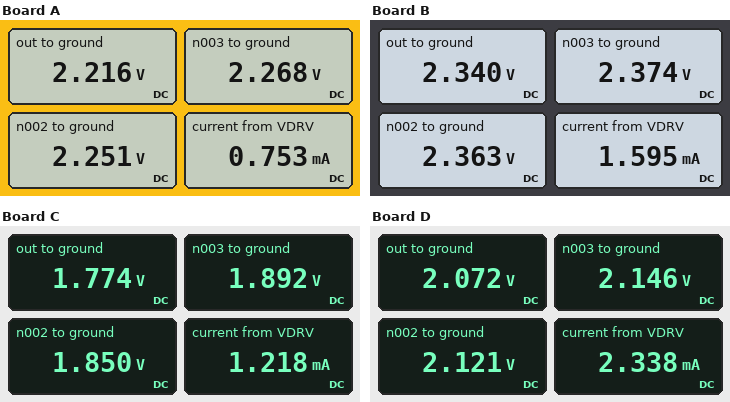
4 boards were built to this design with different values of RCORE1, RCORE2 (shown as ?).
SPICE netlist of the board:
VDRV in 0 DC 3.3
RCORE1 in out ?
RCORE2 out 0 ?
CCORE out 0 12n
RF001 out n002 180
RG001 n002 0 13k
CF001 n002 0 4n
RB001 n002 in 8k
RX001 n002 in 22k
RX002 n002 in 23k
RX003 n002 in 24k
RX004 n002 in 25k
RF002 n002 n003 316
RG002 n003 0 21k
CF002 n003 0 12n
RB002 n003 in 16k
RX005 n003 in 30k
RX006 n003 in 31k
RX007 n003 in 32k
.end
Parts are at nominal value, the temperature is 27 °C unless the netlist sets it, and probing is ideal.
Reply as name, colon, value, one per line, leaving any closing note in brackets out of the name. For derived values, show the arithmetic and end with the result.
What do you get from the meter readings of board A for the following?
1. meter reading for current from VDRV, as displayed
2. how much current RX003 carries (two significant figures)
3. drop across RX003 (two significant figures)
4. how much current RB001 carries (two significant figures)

meter reading for current from VDRV, as displayed: 0.753 mA
how much current RX003 carries: (3.3 V - 2.251 V) / 24 kΩ = 44 µA
drop across RX003: 3.3 V - 2.251 V = 1.0 V
how much current RB001 carries: (3.3 V - 2.251 V) / 8 kΩ = 130 µA
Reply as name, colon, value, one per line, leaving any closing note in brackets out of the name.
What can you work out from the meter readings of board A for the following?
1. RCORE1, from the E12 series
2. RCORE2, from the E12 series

RCORE1, from the E12 series: 3.9 kΩ
RCORE2, from the E12 series: 4.7 kΩ
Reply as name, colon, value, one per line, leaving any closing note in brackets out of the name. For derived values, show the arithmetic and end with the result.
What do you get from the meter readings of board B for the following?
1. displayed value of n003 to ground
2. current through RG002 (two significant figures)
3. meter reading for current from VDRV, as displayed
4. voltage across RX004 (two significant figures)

displayed value of n003 to ground: 2.374 V
current through RG002: (2.374 V) / 21 kΩ = 110 µA
meter reading for current from VDRV, as displayed: 1.595 mA
voltage across RX004: 3.3 V - 2.363 V = 940 mV
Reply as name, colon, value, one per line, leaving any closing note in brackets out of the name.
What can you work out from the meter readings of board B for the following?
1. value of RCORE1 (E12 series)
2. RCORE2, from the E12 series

value of RCORE1: 820 Ω
RCORE2, from the E12 series: 1.8 kΩ
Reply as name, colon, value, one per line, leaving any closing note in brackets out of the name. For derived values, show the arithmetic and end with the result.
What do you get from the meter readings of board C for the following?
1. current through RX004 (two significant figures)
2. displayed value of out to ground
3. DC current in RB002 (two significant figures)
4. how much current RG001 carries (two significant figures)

current through RX004: (3.3 V - 1.85 V) / 25 kΩ = 58 µA
displayed value of out to ground: 1.774 V
DC current in RB002: (3.3 V - 1.892 V) / 16 kΩ = 88 µA
how much current RG001 carries: (1.85 V) / 13 kΩ = 140 µA
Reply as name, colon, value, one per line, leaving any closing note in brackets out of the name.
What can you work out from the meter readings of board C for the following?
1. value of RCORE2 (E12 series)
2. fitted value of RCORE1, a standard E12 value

value of RCORE2: 1.8 kΩ
fitted value of RCORE1, a standard E12 value: 2.7 kΩ
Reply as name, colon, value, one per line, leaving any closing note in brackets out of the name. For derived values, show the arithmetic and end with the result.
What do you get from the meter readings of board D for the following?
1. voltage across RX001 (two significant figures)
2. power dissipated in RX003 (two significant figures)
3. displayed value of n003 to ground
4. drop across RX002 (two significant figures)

voltage across RX001: 3.3 V - 2.121 V = 1.2 V
power dissipated in RX003: (3.3 V - 2.121 V)^2 / 24 kΩ = 58 µW
displayed value of n003 to ground: 2.146 V
drop across RX002: 3.3 V - 2.121 V = 1.2 V
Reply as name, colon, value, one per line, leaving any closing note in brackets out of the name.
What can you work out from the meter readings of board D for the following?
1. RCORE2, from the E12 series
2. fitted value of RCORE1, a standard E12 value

RCORE2, from the E12 series: 1 kΩ
fitted value of RCORE1, a standard E12 value: 680 Ω
